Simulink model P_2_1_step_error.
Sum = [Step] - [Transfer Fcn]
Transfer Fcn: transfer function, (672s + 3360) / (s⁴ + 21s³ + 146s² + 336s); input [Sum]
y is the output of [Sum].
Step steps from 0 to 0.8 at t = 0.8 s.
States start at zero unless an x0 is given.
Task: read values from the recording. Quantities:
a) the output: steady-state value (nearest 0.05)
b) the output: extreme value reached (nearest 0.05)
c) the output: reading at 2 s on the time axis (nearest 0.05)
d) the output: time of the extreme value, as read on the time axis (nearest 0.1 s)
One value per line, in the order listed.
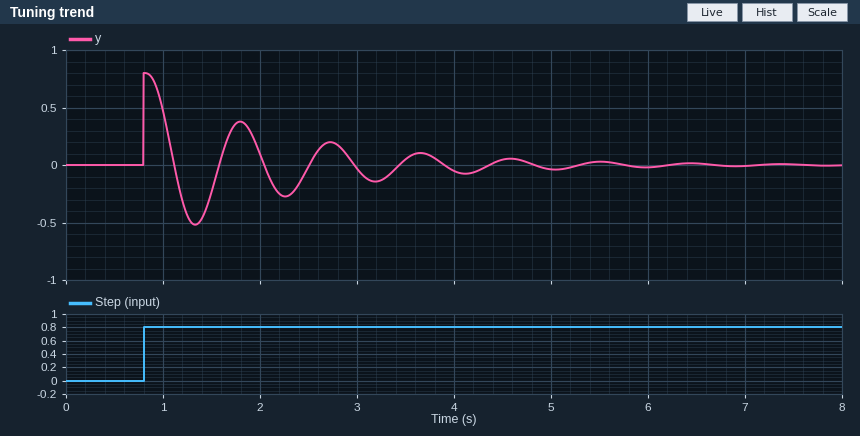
0.00
0.80
0.10
0.8 s
